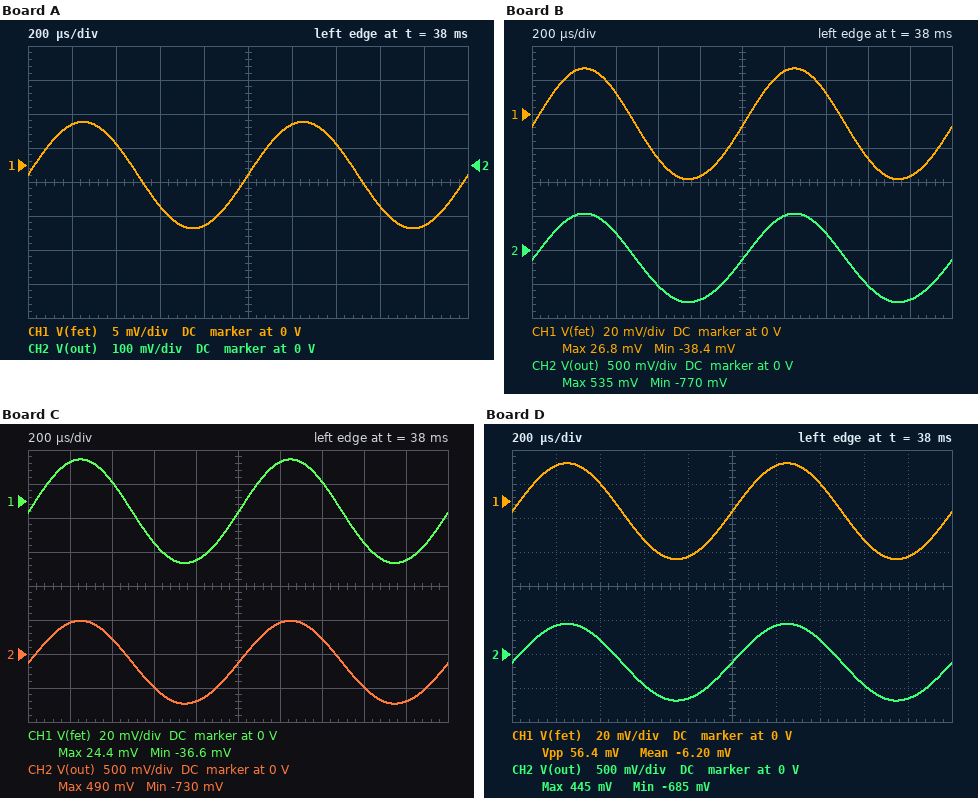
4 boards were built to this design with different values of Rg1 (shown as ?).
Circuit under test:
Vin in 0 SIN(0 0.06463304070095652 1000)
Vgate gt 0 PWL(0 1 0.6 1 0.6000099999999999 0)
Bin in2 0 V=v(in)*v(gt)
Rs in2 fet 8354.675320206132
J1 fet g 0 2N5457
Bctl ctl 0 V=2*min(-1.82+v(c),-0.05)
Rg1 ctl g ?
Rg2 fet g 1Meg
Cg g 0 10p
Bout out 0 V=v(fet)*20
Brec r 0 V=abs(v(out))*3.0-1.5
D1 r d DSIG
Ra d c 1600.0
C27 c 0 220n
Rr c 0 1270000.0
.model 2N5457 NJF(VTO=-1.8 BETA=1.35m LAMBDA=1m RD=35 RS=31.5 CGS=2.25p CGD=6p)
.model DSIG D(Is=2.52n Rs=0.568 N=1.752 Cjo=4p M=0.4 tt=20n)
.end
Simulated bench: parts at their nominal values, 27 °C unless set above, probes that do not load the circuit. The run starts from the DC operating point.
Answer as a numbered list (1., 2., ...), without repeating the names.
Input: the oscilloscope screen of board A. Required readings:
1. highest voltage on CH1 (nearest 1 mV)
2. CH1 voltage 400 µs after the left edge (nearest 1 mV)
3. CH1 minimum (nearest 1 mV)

1. 6 mV
2. 3 mV
3. -9 mV
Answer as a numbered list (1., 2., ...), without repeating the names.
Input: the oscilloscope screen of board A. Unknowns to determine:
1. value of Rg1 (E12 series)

1. 1.5 MΩ
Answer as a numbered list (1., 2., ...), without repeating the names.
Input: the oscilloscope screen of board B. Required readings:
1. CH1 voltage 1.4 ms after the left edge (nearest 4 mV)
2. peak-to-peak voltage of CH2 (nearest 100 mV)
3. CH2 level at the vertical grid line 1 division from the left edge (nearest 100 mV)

1. 12 mV
2. 1.3 V
3. 500 mV
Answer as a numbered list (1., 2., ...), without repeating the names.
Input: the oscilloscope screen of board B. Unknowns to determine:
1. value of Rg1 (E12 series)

1. 560 kΩ
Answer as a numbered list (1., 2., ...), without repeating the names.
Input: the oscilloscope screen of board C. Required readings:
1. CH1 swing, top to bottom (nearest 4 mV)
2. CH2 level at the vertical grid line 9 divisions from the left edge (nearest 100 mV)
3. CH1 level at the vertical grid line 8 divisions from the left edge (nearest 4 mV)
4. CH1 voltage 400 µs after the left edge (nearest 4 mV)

1. 60 mV
2. -700 mV
3. -24 mV
4. 12 mV
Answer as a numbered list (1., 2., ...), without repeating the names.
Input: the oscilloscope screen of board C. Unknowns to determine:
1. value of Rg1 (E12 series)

1. 680 kΩ
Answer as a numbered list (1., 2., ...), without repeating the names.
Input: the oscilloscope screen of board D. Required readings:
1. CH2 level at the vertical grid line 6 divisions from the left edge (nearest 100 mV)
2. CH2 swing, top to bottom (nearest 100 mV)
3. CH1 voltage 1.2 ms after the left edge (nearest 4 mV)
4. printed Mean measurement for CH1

1. 400 mV
2. 1.1 V
3. 20 mV
4. -6.20 mV
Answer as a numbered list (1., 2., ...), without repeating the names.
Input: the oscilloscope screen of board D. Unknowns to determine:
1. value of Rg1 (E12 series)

1. 820 kΩ
